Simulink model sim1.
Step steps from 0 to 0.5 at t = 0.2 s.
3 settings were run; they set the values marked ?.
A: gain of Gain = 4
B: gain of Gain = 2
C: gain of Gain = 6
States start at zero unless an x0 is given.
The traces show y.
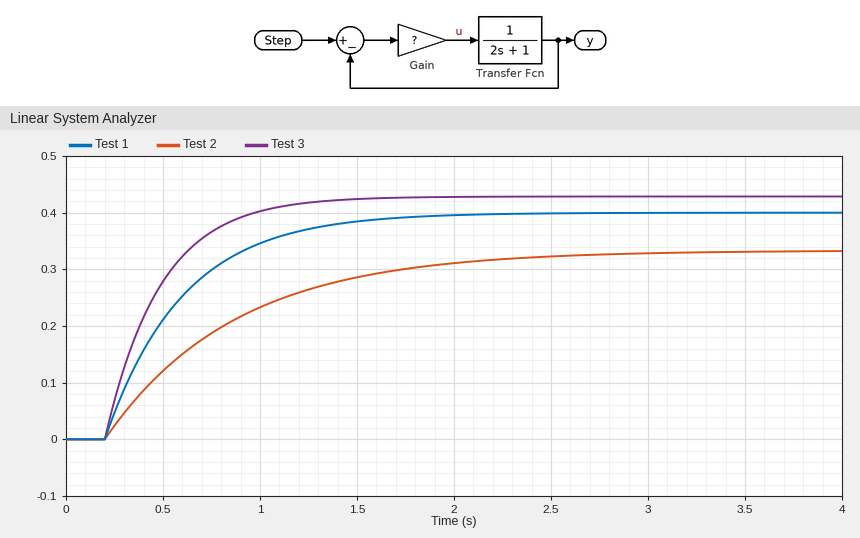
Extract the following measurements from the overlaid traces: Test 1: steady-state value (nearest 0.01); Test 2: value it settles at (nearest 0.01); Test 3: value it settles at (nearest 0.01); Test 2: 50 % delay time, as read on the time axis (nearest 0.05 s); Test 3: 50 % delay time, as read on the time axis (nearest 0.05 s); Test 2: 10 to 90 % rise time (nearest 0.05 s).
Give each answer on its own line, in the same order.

0.40
0.33
0.43
0.65 s
0.40 s
1.45 s
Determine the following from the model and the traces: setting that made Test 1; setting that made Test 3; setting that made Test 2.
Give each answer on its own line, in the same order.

A
C
B
